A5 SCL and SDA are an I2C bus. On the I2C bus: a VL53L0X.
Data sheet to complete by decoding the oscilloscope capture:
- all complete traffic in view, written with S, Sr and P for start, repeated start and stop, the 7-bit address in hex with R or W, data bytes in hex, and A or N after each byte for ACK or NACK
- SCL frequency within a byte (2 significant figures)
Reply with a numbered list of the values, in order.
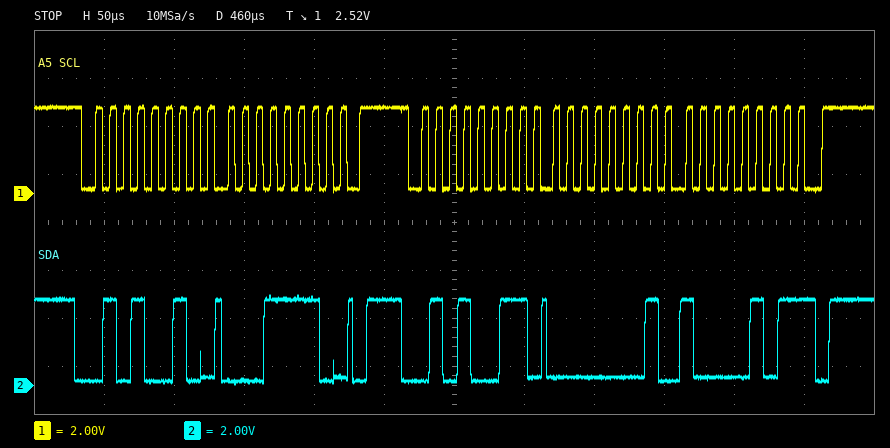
1. S 29W A 1E A P S 29R A 01 A 85 N P
2. 100 kHz
